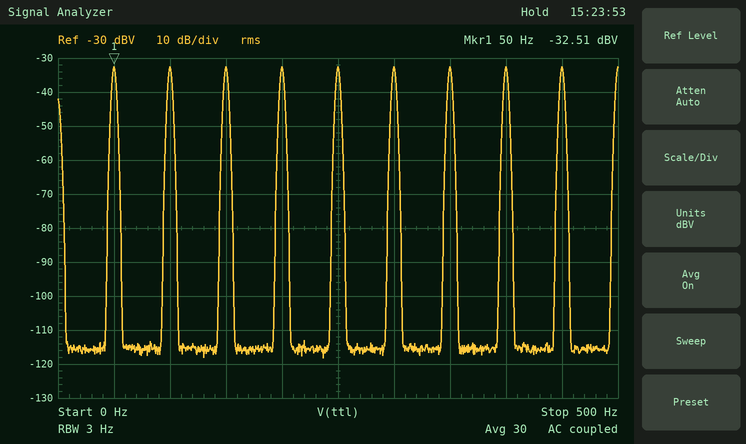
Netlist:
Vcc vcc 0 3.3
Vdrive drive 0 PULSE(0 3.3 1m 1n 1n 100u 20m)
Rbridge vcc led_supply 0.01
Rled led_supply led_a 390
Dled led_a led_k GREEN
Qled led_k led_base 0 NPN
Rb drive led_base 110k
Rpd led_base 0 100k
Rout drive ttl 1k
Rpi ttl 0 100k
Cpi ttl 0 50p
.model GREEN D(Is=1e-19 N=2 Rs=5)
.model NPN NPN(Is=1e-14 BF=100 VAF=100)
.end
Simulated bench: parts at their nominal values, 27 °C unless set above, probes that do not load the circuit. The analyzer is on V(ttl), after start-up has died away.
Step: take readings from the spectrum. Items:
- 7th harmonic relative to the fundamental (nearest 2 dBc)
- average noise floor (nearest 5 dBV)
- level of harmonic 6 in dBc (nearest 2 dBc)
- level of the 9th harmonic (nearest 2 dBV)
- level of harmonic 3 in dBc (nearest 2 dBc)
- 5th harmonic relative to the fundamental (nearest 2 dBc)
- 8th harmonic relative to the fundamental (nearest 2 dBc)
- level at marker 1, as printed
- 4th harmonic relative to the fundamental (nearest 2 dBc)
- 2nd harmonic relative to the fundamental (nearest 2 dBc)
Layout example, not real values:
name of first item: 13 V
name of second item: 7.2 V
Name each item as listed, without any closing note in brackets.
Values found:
7th harmonic relative to the fundamental: 0 dBc
average noise floor: -115 dBV
level of harmonic 6 in dBc: 0 dBc
level of the 9th harmonic: -32 dBV
level of harmonic 3 in dBc: 0 dBc
5th harmonic relative to the fundamental: 0 dBc
8th harmonic relative to the fundamental: 0 dBc
level at marker 1, as printed: -32.51 dBV
4th harmonic relative to the fundamental: 0 dBc
2nd harmonic relative to the fundamental: 0 dBc
